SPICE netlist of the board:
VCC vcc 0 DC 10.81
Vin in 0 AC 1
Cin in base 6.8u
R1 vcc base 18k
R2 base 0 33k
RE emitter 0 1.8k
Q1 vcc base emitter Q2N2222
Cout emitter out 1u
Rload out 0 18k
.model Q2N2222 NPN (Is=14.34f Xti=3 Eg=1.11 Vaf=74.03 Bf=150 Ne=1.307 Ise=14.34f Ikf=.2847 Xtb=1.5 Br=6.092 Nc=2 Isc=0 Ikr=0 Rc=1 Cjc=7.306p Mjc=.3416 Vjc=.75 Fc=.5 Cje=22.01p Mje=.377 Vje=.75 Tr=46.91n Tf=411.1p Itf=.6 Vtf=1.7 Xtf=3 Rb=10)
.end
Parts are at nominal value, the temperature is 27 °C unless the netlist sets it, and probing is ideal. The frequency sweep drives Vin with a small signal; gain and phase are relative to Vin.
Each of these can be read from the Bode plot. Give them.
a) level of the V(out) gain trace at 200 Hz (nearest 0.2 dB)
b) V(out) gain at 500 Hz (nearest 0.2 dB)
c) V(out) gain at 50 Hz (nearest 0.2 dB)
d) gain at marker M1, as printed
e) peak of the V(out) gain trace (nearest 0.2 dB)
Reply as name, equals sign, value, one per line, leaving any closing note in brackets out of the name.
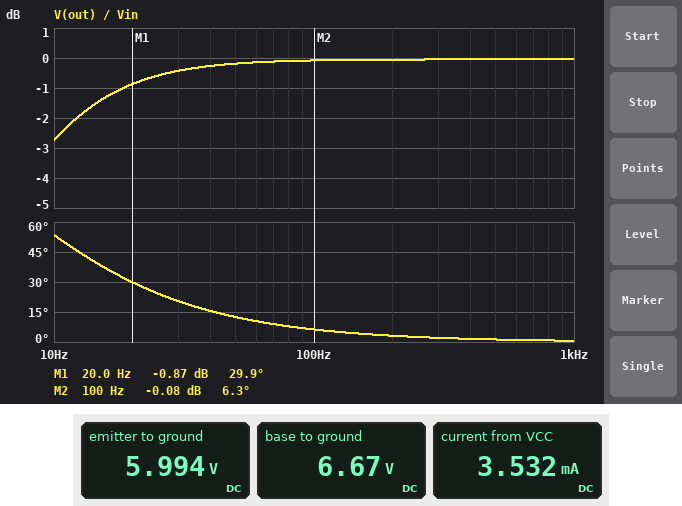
level of the V(out) gain trace at 200 Hz = 0 dB
V(out) gain at 500 Hz = 0 dB
V(out) gain at 50 Hz = -0.2 dB
gain at marker M1, as printed = -0.87 dB
peak of the V(out) gain trace = 0 dB
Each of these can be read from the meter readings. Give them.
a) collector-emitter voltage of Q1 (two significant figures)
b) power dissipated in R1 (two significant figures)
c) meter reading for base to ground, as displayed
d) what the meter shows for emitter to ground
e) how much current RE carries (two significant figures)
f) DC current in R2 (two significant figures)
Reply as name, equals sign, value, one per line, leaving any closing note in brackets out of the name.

collector-emitter voltage of Q1 = 4.8 V
power dissipated in R1 = 950 µW
meter reading for base to ground, as displayed = 6.67 V
what the meter shows for emitter to ground = 5.994 V
how much current RE carries = 3.3 mA
DC current in R2 = 200 µA
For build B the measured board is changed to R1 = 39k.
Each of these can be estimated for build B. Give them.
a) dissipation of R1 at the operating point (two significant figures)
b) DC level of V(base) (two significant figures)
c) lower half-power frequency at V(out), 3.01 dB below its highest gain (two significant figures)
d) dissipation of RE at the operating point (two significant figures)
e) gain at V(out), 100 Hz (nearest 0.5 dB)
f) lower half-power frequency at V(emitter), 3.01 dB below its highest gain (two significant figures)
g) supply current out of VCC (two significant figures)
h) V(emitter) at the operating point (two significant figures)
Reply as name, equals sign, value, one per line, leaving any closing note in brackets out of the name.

dissipation of R1 at the operating point = 980 µW
DC level of V(base) = 4.6 V
lower half-power frequency at V(out), 3.01 dB below its highest gain = 9.1 Hz
dissipation of RE at the operating point = 8.7 mW
gain at V(out), 100 Hz = 0 dB
lower half-power frequency at V(emitter), 3.01 dB below its highest gain = 1.4 Hz
supply current out of VCC = 2.3 mA
V(emitter) at the operating point = 4.0 V
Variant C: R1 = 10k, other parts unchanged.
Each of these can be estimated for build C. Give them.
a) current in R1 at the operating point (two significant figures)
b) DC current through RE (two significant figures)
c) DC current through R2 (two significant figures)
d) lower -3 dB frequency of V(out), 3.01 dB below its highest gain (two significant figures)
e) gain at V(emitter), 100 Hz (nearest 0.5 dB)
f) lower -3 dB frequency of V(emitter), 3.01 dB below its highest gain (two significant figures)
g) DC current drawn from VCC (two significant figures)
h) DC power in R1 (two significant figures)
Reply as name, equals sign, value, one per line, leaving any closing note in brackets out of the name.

current in R1 at the operating point = 280 µA
DC current through RE = 4.1 mA
DC current through R2 = 240 µA
lower -3 dB frequency of V(out), 3.01 dB below its highest gain = 9.8 Hz
gain at V(emitter), 100 Hz = 0 dB
lower -3 dB frequency of V(emitter), 3.01 dB below its highest gain = 3.2 Hz
DC current drawn from VCC = 4.3 mA
DC power in R1 = 770 µW
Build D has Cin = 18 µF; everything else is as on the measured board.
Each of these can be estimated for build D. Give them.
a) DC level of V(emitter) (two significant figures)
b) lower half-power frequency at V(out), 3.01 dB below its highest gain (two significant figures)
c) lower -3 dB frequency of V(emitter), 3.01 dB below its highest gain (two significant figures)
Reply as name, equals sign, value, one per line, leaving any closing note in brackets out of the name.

DC level of V(emitter) = 6.0 V
lower half-power frequency at V(out), 3.01 dB below its highest gain = 8.9 Hz
lower -3 dB frequency of V(emitter), 3.01 dB below its highest gain = 800 mHz
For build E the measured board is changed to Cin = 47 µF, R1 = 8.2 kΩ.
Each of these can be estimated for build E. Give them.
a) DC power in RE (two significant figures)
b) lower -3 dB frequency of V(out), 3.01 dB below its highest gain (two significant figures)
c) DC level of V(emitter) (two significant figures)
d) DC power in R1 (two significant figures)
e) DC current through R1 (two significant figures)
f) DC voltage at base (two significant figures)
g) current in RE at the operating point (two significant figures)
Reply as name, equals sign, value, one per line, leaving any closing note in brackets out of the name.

DC power in RE = 33 mW
lower -3 dB frequency of V(out), 3.01 dB below its highest gain = 8.9 Hz
DC level of V(emitter) = 7.7 V
DC power in R1 = 700 µW
DC current through R1 = 290 µA
DC voltage at base = 8.4 V
current in RE at the operating point = 4.3 mA
